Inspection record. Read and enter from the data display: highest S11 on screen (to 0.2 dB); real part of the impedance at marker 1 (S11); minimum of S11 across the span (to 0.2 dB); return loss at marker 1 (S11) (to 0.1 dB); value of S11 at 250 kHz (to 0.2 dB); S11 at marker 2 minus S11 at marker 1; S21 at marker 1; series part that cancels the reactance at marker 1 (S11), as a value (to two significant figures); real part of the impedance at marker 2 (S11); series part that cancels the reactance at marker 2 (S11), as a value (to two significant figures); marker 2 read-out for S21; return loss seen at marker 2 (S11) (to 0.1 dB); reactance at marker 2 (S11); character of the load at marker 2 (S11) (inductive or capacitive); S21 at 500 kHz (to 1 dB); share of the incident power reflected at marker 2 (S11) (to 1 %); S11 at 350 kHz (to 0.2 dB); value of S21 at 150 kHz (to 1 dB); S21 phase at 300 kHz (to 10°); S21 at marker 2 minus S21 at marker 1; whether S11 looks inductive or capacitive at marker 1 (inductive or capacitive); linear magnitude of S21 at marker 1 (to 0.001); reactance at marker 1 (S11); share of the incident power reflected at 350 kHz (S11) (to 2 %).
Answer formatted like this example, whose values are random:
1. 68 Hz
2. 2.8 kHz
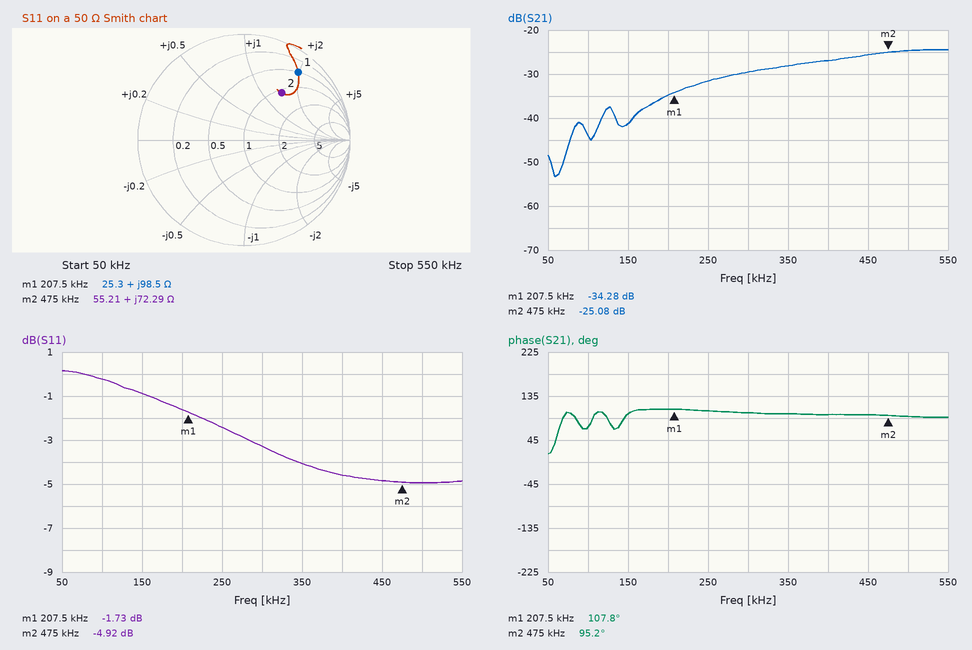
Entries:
1. 0.2 dB
2. 25.3 Ω
3. -5.0 dB
4. 1.7 dB
5. -2.4 dB
6. -3.19 dB
7. -34.28 dB
8. 7.8 nF
9. 55.21 Ω
10. 4.6 nF
11. -25.08 dB
12. 4.9 dB
13. +72.29 Ω
14. inductive
15. -25 dB
16. 32 %
17. -4.0 dB
18. -41 dB
19. 100°
20. 9.20 dB
21. inductive
22. 0.019
23. +98.5 Ω
24. 40 %
